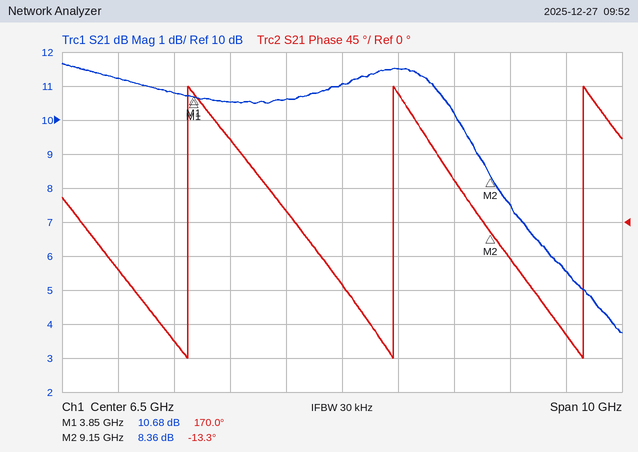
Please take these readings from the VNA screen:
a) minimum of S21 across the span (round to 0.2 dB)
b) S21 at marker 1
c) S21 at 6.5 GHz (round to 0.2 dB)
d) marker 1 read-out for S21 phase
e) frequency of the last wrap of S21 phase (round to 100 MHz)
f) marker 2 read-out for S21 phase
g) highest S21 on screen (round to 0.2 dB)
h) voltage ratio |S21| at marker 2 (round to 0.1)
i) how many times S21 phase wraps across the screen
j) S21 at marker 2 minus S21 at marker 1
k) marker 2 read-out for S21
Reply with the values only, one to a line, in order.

3.8 dB
10.68 dB
11.0 dB
170.0°
10.8 GHz
-13.3°
11.6 dB
2.6
3
-2.32 dB
8.36 dB
